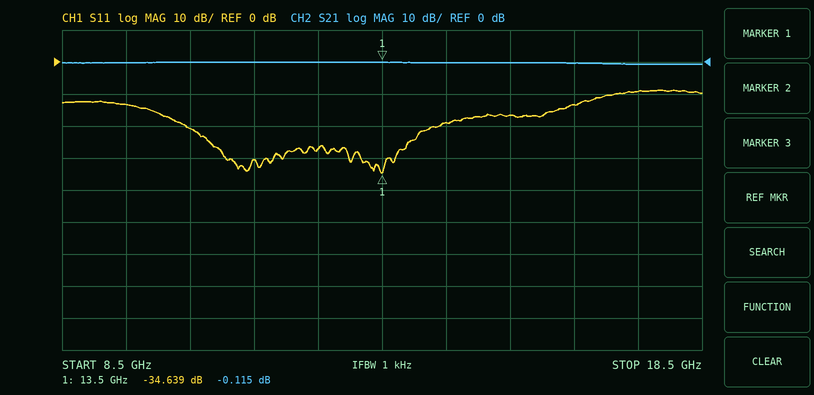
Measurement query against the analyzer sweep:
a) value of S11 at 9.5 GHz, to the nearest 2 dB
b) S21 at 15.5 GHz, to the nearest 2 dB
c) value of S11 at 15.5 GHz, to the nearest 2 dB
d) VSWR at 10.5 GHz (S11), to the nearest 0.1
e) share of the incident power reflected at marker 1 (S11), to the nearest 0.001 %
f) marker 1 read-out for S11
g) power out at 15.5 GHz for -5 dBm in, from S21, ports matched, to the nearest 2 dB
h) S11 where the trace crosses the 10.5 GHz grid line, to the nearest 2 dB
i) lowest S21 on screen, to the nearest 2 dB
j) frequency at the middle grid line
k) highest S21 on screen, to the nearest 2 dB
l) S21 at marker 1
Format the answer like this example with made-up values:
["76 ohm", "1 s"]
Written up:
["-14 dB", "0 dB", "-16 dB", "1.2", "0.034 %", "-34.639 dB", "-6 dBm", "-20 dB", "0 dB", "13.5 GHz", "0 dB", "-0.115 dB"]
